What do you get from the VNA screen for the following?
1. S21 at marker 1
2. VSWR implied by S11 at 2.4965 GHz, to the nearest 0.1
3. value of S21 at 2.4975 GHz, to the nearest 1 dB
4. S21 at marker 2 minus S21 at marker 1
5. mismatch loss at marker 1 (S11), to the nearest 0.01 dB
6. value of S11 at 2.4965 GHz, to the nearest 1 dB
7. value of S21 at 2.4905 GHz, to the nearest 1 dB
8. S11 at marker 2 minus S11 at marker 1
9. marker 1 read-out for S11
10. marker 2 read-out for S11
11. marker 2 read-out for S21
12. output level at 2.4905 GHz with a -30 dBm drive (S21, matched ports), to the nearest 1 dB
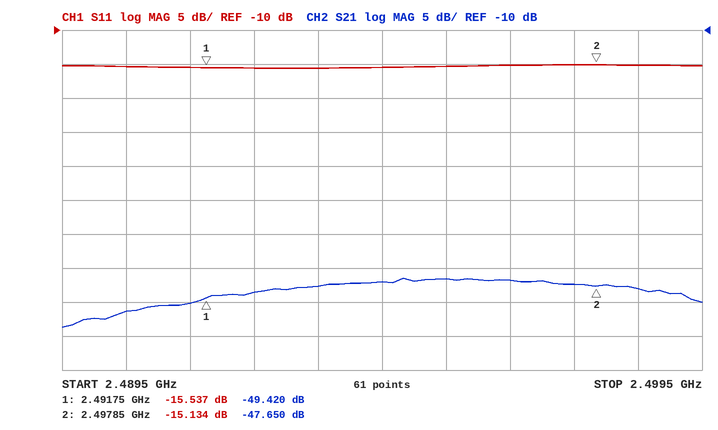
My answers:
-49.420 dB
1.4
-47 dB
1.770 dB
0.12 dB
-15 dB
-51 dB
0.403 dB
-15.537 dB
-15.134 dB
-47.650 dB
-81 dBm
